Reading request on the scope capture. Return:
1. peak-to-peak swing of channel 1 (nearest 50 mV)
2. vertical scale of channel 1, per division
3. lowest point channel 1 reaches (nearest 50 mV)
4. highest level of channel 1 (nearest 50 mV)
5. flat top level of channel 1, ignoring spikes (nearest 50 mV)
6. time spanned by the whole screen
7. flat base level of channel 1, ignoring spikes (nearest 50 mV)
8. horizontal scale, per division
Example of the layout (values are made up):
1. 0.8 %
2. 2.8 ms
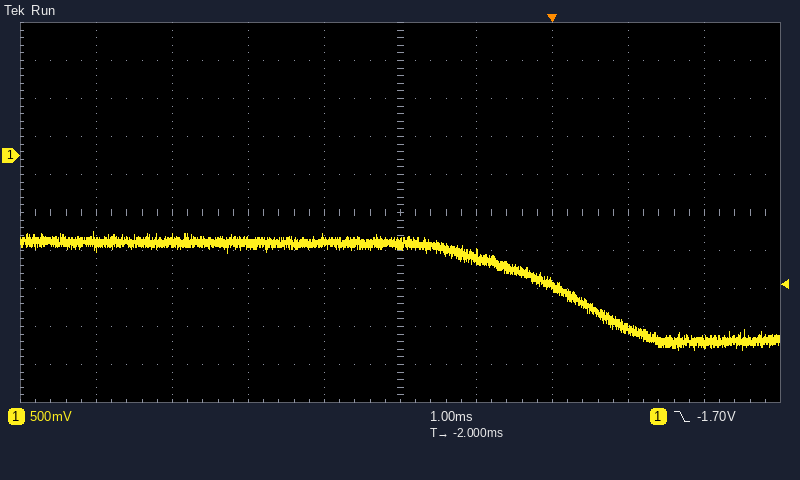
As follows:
1. 1.55 V
2. 500 mV
3. -2.55 V
4. -1.00 V
5. -1.15 V
6. 10 ms
7. -2.45 V
8. 1 ms
